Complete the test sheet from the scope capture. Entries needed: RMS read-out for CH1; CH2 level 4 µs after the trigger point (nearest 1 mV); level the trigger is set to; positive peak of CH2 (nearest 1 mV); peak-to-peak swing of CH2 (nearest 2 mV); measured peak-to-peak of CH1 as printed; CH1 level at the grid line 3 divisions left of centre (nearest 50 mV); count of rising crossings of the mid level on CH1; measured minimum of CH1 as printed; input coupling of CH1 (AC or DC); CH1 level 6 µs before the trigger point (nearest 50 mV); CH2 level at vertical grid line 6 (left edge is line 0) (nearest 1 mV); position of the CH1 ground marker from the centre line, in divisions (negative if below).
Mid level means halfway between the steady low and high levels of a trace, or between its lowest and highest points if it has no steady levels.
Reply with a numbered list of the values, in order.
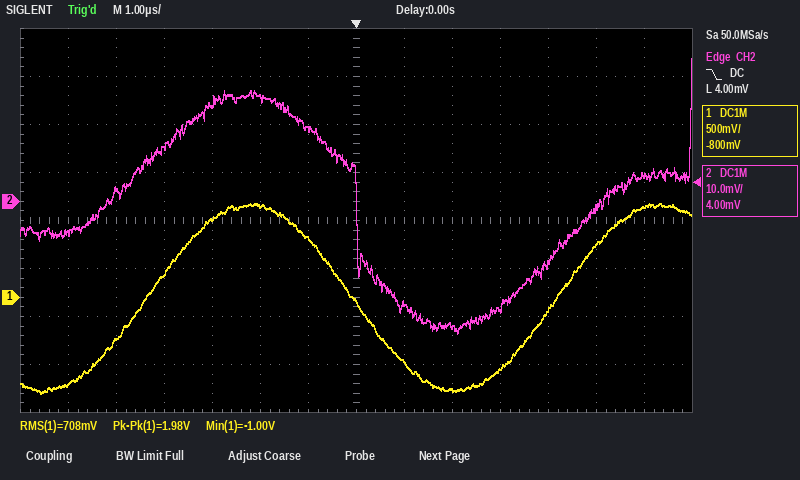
1. 708 mV
2. -13 mV
3. 4.00 mV
4. 30 mV
5. 58 mV
6. 1.98 V
7. 800 mV
8. 2
9. -1.00 V
10. DC
11. -900 mV
12. 15 mV
13. -1.6 div
